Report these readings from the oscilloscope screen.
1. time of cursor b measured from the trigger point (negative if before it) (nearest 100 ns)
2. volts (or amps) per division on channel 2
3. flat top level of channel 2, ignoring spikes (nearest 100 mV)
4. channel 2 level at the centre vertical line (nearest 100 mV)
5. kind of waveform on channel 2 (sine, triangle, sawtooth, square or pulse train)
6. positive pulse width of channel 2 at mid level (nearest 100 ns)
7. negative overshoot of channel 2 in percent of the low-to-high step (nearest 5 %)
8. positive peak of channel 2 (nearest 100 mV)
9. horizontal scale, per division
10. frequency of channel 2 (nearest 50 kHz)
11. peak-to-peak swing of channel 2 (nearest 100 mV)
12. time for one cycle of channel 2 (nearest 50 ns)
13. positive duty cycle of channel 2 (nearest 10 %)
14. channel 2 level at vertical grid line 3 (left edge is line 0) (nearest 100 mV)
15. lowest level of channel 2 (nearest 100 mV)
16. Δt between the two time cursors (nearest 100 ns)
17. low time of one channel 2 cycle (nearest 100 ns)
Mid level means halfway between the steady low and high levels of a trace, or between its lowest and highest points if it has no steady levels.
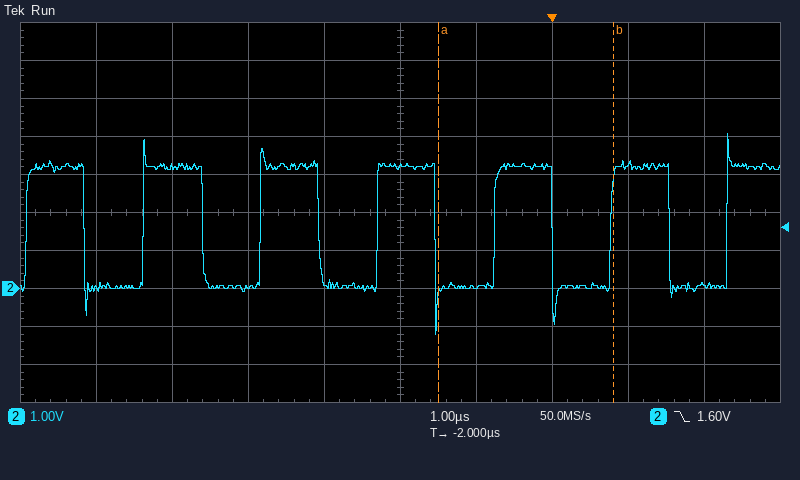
+800 ns
1 V
3.2 V
3.2 V
square
800 ns
40 %
4.1 V
1 µs
650 kHz
5.3 V
1.55 µs
50 %
0.0 V
-1.2 V
2.3 µs
800 ns
